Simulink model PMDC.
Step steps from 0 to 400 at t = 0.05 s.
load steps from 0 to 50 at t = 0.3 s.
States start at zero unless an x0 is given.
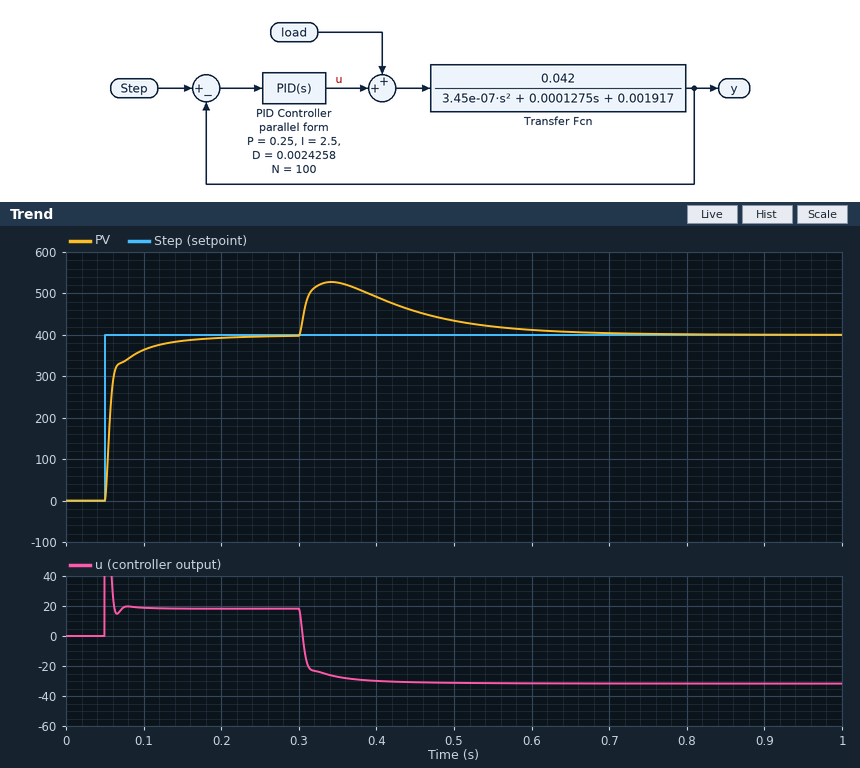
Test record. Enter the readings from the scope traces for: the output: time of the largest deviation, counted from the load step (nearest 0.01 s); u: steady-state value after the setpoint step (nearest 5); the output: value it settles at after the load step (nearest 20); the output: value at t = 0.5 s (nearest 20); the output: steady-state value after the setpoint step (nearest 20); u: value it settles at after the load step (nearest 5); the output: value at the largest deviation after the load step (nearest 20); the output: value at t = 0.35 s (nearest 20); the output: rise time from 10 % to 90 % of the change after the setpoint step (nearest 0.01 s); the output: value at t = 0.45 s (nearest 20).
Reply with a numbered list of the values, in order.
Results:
1. 0.04 s
2. 20
3. 400
4. 440
5. 400
6. -30
7. 520
8. 520
9. 0.04 s
10. 460
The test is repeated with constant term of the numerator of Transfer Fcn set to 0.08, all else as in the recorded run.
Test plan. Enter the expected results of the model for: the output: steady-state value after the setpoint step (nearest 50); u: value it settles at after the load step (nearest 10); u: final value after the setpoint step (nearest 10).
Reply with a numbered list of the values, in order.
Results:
1. 400
2. -40
3. 10
